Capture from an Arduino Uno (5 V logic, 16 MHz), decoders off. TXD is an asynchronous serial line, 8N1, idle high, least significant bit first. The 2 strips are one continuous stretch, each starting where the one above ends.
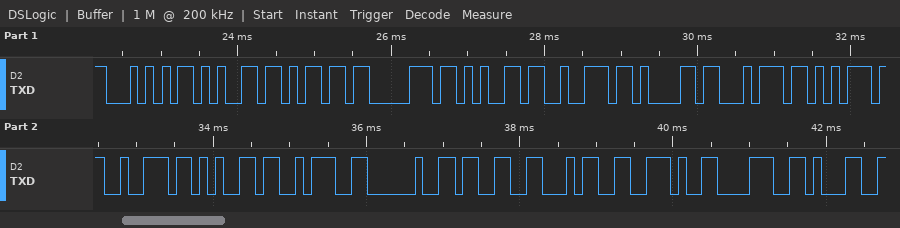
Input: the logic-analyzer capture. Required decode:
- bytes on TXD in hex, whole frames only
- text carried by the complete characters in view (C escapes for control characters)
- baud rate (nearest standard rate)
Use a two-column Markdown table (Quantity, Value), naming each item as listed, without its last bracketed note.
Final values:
| Quantity | Value |
|---|---|
| bytes on TXD in hex, whole frames only | 54 65 6D 70 65 72 61 74 75 72 65 3A 20 33 34 2E 38 31 |
| text carried by the complete characters in view | "Temperature: 34.81" |
| baud rate | 9600 baud |
